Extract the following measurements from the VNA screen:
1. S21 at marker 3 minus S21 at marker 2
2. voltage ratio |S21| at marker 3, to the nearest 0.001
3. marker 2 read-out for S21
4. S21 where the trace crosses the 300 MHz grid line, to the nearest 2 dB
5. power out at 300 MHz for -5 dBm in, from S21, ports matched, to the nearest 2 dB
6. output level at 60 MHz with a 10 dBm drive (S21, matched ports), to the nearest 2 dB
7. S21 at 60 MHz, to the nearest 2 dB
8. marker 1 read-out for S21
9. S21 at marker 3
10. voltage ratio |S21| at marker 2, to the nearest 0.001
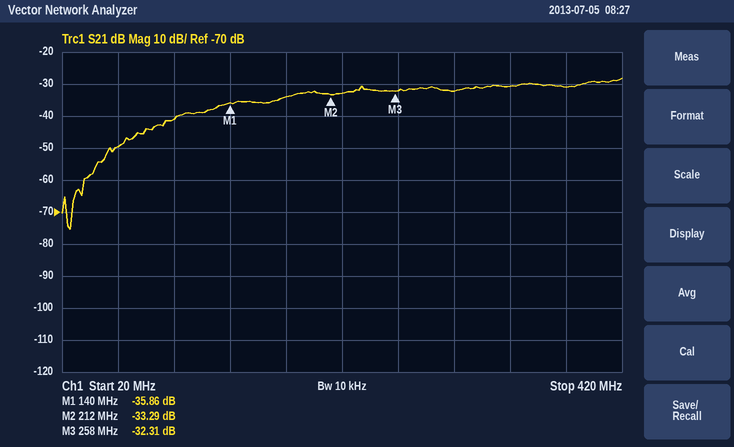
0.98 dB
0.024
-33.29 dB
-32 dB
-38 dBm
-40 dBm
-50 dB
-35.86 dB
-32.31 dB
0.022
